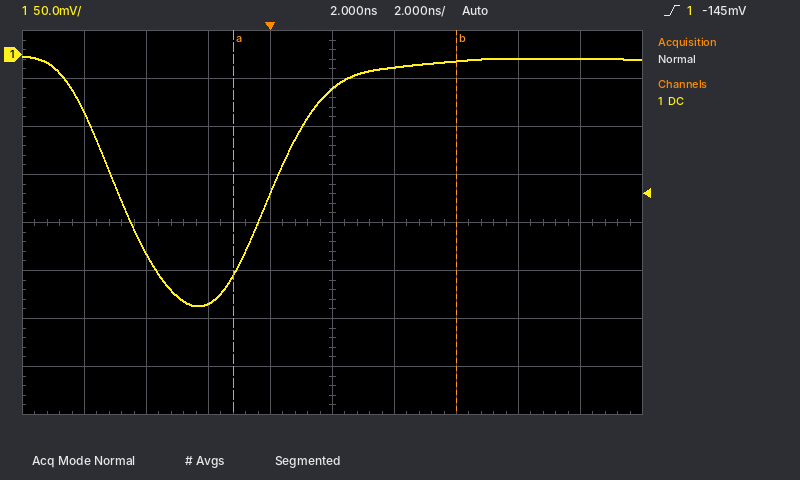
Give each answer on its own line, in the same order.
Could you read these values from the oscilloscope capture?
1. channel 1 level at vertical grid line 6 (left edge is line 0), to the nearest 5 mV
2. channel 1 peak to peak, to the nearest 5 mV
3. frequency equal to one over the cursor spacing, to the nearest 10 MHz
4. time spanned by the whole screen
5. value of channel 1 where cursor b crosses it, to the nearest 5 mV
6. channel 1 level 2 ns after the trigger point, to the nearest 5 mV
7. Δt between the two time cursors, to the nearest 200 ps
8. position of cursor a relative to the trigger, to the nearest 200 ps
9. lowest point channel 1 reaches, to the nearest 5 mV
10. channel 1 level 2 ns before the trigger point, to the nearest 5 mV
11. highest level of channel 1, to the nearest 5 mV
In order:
-15 mV
260 mV
140 MHz
20 ns
-5 mV
-35 mV
7.2 ns
-1.2 ns
-260 mV
-260 mV
0 mV
